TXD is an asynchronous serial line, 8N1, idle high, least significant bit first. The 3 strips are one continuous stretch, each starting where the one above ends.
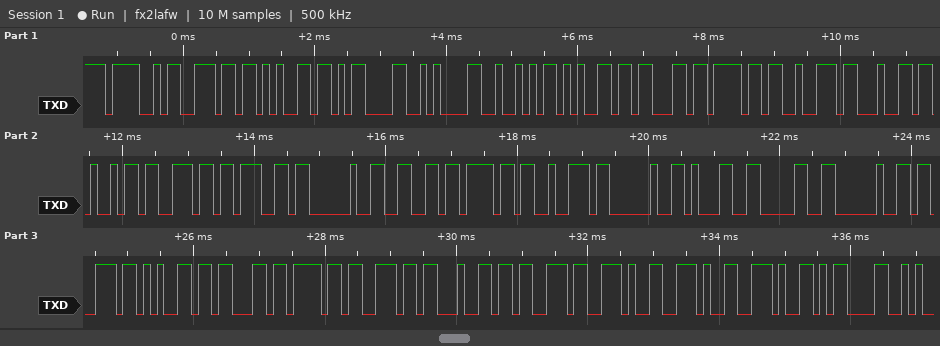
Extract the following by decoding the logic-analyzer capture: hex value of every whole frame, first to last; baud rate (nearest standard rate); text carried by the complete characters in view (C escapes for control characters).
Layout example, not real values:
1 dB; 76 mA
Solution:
0x4F 0x6E 0x65 0x0D 0x0A 0x52 0x65 0x63 0x6F 0x72 0x64 0x69 0x6E 0x67 0x20 0x66 0x6F 0x72 0x20 0x31 0x30 0x20 0x73 0x65 0x63 0x6F 0x6E 0x64 0x73 0x2E 0x2E 0x2E 0x0D; 9600 baud; "One\r\nRecording for 10 seconds...\r"
